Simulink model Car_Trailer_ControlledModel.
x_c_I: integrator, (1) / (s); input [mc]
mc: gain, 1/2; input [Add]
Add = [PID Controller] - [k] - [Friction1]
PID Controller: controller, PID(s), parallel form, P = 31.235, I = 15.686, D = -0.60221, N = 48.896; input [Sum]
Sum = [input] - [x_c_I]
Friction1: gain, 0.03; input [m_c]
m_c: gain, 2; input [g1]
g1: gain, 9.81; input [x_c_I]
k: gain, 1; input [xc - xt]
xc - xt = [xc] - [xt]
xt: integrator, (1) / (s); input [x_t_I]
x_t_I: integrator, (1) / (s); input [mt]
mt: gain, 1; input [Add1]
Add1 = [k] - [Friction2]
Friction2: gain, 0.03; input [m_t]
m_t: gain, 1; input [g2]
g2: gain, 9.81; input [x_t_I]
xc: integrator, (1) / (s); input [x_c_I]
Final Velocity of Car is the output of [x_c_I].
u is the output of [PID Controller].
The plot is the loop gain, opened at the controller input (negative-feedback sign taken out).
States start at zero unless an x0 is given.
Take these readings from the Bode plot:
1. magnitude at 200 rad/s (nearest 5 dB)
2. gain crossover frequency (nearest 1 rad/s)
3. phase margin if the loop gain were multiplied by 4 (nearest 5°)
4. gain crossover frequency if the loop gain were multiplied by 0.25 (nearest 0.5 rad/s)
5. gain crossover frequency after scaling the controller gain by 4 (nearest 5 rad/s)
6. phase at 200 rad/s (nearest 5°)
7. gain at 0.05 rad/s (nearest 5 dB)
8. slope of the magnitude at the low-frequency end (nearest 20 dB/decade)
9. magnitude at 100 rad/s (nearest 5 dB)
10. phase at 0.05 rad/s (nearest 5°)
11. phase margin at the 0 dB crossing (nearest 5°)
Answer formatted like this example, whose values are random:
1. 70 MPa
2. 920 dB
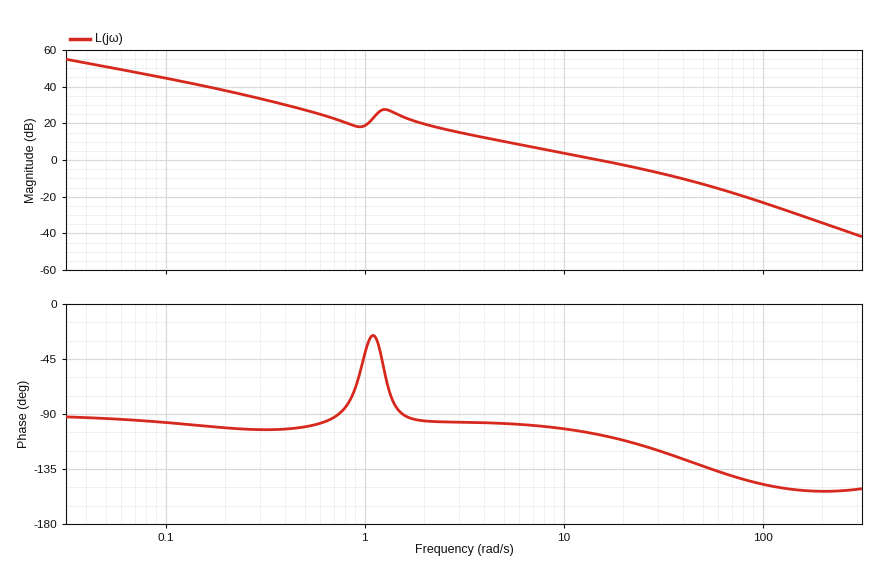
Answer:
1. -35 dB
2. 15 rad/s
3. 50°
4. 4.0 rad/s
5. 45 rad/s
6. -155°
7. 50 dB
8. -20 dB/decade
9. -25 dB
10. -95°
11. 75°
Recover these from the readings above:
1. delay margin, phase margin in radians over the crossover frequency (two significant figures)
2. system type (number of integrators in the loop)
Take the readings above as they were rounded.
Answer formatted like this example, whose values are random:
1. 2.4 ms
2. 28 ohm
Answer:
1. 0.087 s
2. 1
